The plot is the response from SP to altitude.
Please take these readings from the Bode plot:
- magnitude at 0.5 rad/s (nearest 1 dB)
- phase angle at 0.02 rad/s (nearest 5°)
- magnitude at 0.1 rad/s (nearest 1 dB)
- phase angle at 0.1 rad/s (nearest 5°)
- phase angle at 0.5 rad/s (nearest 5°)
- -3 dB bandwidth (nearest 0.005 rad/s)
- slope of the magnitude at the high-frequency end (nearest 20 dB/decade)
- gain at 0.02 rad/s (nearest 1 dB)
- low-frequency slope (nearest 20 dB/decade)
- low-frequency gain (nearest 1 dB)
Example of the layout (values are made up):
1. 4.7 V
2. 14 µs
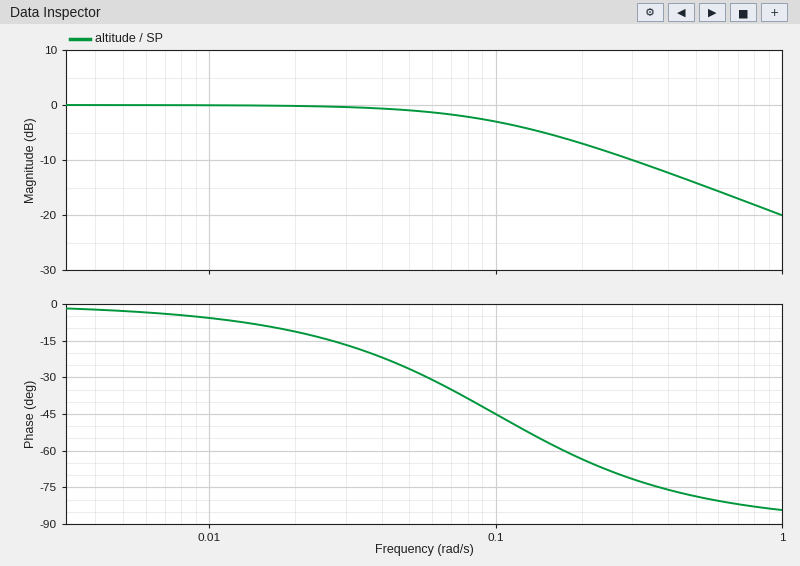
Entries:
1. -14 dB
2. -10°
3. -3 dB
4. -45°
5. -80°
6. 0.100 rad/s
7. -20 dB/decade
8. 0 dB
9. 0 dB/decade
10. 0 dB
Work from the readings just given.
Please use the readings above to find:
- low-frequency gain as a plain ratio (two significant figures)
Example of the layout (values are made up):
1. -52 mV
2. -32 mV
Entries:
1. 1.0
